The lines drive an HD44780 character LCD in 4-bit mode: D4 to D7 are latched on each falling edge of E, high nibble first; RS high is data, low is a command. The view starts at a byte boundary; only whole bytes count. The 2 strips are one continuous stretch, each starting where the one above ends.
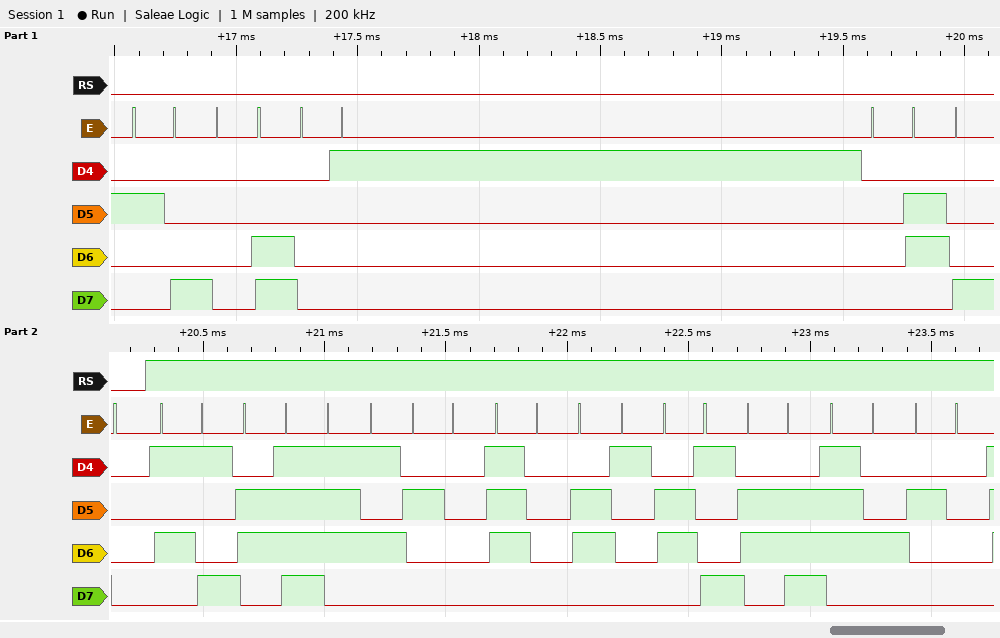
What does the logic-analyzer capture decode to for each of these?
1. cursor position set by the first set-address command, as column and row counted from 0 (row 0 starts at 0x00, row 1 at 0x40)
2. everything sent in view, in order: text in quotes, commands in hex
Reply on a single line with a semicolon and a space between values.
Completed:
column 0, row 0; 0x28 0x0C 0x01 0x06 0x80 "You paint "
